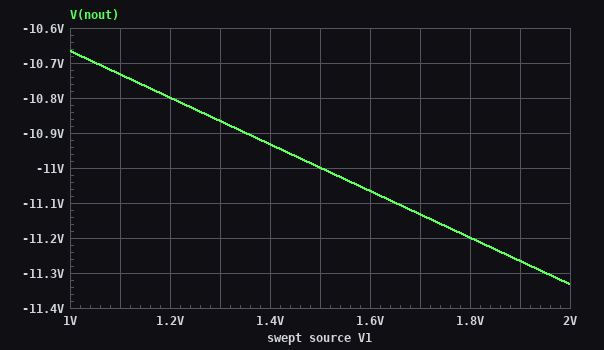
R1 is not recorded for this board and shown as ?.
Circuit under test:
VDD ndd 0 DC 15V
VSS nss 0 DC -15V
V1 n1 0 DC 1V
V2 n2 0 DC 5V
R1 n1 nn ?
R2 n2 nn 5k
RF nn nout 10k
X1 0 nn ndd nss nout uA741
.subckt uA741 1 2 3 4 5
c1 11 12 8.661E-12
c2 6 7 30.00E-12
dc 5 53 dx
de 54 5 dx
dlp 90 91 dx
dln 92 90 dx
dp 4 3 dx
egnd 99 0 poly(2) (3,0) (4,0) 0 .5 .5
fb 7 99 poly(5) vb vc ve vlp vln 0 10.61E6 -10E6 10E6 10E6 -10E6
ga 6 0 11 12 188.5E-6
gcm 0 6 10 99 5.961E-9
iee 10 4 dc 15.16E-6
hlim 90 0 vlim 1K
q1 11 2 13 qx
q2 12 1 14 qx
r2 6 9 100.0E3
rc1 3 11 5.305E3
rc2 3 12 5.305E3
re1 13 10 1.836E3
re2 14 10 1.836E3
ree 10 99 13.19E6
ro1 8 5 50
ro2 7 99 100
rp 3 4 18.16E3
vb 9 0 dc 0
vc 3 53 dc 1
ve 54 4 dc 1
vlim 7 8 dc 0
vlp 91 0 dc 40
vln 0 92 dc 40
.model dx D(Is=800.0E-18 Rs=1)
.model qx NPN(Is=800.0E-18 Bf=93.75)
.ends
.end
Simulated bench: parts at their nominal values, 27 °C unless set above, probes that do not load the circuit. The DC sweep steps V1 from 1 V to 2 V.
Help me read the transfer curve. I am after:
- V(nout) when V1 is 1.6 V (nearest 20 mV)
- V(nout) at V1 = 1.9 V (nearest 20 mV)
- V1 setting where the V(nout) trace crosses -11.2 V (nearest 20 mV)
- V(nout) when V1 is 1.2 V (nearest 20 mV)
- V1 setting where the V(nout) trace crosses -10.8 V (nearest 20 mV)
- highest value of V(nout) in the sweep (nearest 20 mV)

-11.06 V
-11.26 V
1.80 V
-10.80 V
1.20 V
-10.66 V
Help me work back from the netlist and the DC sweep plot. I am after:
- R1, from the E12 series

15 kΩ
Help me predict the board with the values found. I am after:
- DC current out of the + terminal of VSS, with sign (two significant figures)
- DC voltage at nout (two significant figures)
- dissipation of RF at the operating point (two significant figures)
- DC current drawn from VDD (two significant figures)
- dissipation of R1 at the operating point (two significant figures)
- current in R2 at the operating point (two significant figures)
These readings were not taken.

-1.7 mA
-11 V
11 mW
1.7 mA
67 µW
1.0 mA
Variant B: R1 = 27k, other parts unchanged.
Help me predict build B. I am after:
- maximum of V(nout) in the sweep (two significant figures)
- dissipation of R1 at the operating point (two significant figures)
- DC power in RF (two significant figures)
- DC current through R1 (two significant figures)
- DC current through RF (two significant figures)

-10 V
37 µW
11 mW
37 µA
1.0 mA
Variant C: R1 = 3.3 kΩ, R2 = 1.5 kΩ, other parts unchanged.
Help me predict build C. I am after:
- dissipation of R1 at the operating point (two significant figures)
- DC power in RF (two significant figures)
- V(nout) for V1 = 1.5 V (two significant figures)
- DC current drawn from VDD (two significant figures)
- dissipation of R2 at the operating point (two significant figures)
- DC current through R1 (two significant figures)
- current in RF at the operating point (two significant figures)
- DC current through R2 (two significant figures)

320 µW
28 mW
-15 V
1.7 mA
5.9 mW
310 µA
1.7 mA
2.0 mA
